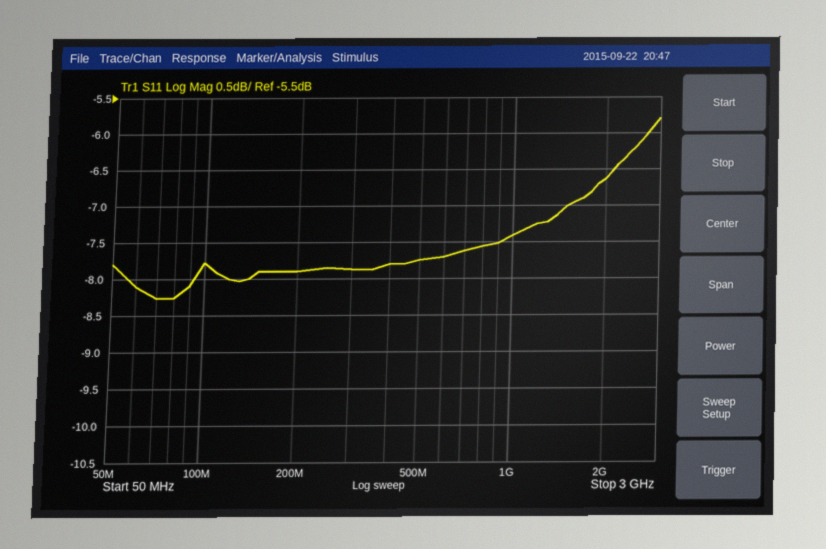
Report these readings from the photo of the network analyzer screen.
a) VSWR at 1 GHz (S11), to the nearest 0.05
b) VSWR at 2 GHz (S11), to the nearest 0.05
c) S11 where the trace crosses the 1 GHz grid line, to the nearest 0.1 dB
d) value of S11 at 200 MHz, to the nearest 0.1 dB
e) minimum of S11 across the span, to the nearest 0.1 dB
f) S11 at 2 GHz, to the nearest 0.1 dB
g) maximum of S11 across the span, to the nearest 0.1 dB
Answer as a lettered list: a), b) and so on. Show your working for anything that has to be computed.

a) |Γ| = 10^(-7.4/20) = 0.4266; VSWR = (1 + 0.4266)/(1 − 0.4266) ≈ 2.49, so 2.50 to the nearest 0.05
b) |Γ| = 10^(-6.6/20) = 0.4677; VSWR = (1 + 0.4677)/(1 − 0.4677) ≈ 2.76, so 2.75 to the nearest 0.05
c) -7.4 dB
d) -7.9 dB
e) -8.3 dB
f) -6.6 dB
g) -5.8 dB
